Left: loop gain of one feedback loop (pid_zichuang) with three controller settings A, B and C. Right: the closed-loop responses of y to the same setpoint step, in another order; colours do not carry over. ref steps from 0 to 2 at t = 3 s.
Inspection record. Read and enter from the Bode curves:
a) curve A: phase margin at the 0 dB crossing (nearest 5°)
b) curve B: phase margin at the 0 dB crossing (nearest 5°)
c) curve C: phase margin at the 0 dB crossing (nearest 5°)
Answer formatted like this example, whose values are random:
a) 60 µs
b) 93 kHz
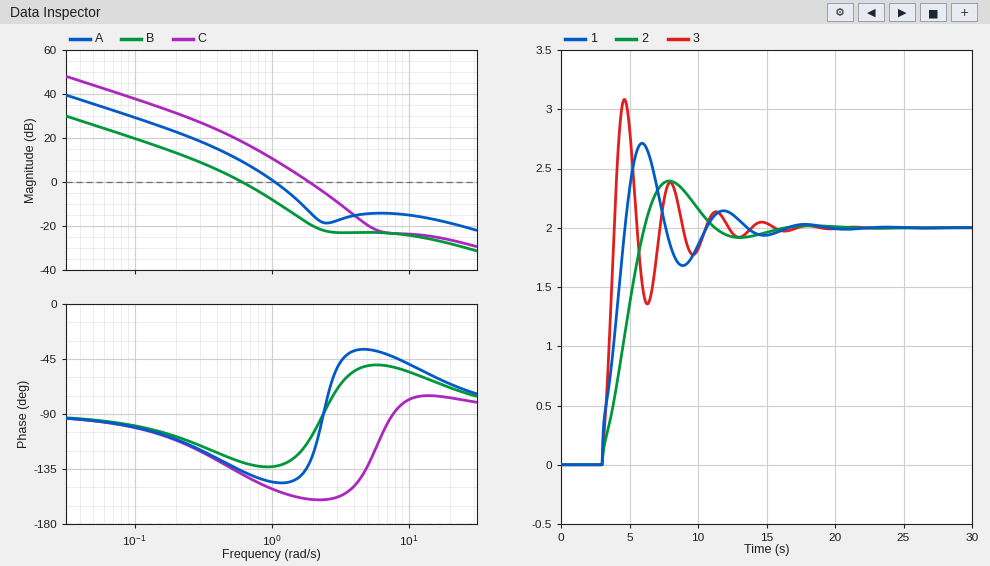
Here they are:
a) 35°
b) 50°
c) 20°
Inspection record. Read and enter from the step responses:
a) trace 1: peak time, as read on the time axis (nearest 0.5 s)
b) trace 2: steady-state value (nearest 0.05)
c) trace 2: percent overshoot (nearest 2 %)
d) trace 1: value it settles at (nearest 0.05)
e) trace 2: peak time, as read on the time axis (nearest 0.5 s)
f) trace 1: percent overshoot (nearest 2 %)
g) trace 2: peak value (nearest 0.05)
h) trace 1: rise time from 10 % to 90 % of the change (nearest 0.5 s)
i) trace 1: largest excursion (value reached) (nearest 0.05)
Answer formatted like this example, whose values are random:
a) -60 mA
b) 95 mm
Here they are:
a) 6.0 s
b) 2.00
c) 20 %
d) 2.00
e) 8.0 s
f) 36 %
g) 2.40
h) 1.5 s
i) 2.70
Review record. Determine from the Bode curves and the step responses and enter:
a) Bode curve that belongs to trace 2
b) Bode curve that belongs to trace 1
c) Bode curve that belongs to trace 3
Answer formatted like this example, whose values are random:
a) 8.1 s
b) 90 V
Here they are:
a) B
b) A
c) C
